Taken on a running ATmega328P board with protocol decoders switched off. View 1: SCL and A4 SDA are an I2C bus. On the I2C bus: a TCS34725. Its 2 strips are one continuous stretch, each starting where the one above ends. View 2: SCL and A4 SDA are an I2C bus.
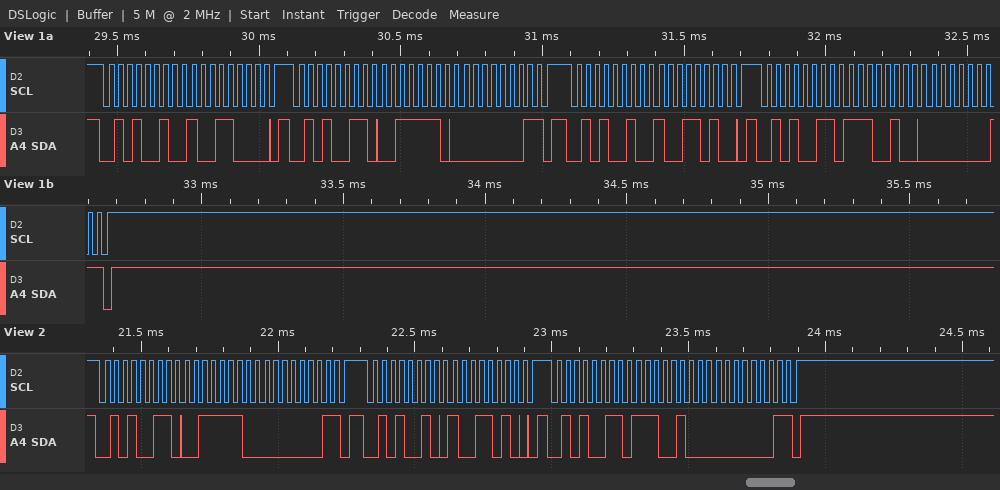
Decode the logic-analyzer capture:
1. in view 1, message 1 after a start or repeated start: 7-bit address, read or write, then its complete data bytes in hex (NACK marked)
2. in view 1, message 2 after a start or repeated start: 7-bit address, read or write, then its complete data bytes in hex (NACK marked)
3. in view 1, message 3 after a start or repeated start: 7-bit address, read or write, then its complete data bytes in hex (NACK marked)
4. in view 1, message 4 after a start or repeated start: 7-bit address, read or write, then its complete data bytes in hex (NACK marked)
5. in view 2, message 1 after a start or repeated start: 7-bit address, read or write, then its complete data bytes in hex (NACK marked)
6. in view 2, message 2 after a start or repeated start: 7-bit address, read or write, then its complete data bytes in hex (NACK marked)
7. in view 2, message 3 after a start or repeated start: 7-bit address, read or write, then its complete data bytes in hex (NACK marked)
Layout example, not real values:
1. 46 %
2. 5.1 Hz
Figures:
1. 0x29 write: 98
2. 0x29 read: 3E 01 NACK
3. 0x29 write: 9A
4. 0x29 read: E4 01 NACK
5. 0x29 read: 3E 01 NACK
6. 0x29 write: 9A
7. 0x29 read: E4 01 NACK
